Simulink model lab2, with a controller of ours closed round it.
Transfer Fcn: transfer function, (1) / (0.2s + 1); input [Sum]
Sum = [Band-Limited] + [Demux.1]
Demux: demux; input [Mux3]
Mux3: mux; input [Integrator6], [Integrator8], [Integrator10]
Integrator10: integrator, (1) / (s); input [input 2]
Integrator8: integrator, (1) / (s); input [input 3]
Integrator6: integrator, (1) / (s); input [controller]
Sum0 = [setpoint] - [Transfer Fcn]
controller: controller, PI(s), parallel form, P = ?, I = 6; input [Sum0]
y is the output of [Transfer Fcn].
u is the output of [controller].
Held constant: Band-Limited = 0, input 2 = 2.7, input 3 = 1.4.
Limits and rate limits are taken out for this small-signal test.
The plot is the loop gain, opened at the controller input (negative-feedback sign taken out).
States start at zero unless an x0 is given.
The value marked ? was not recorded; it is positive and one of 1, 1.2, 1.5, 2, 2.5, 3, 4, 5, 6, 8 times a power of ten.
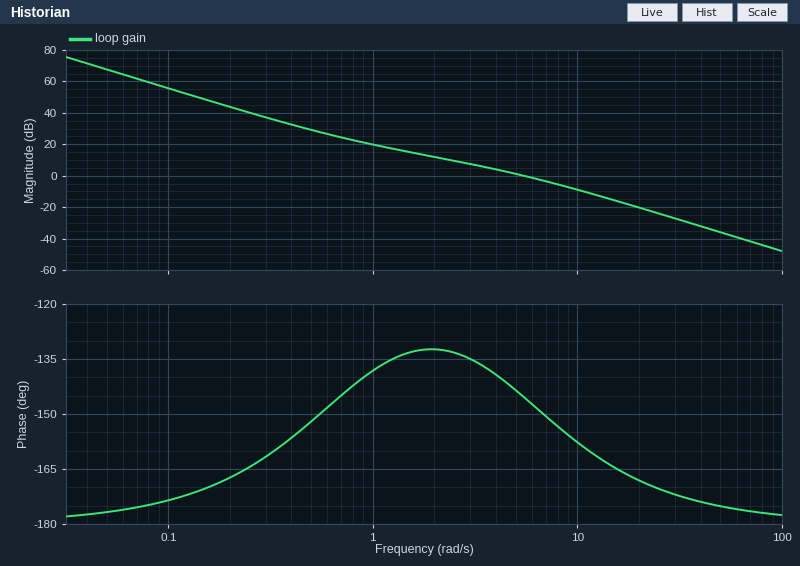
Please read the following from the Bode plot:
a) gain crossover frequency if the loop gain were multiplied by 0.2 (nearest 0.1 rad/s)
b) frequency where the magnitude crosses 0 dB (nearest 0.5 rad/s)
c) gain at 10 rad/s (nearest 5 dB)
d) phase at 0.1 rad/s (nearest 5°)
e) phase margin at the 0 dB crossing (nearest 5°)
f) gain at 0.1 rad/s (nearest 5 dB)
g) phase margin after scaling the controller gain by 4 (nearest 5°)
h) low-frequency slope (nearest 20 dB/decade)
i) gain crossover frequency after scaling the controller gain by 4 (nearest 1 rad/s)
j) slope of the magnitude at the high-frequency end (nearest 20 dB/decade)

1.7 rad/s
5.5 rad/s
-10 dB
-175°
35°
55 dB
20°
-40 dB/decade
12 rad/s
-40 dB/decade
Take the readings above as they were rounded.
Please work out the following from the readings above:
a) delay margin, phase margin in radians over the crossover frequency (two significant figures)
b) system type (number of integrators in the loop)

0.11 s
2
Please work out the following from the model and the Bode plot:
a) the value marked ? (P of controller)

8
